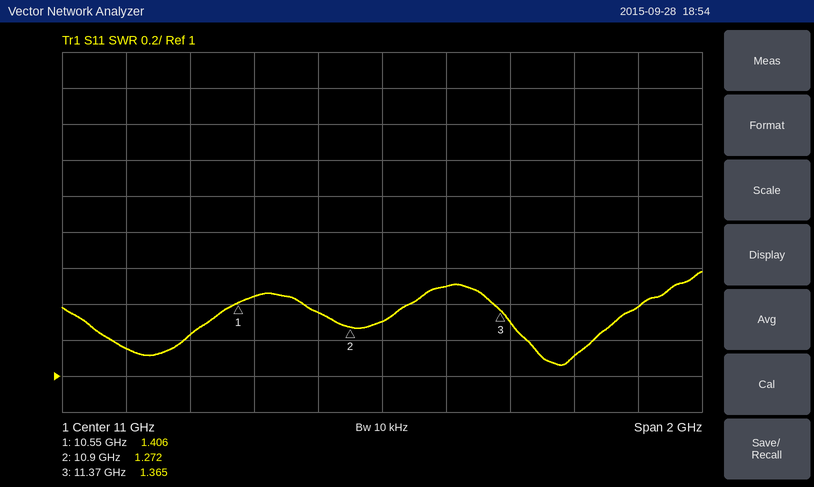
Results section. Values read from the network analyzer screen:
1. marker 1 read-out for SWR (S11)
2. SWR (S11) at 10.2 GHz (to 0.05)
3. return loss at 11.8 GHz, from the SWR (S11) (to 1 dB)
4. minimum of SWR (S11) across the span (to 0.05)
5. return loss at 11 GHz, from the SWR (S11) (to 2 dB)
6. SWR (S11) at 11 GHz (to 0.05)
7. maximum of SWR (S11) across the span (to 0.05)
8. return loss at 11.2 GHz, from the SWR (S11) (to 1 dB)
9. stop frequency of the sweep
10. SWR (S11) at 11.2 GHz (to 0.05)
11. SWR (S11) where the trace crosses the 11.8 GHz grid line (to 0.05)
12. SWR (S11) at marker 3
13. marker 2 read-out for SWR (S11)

1.406
1.15
16 dB
1.05
18 dB
1.30
1.60
14 dB
12 GHz
1.50
1.40
1.365
1.272
